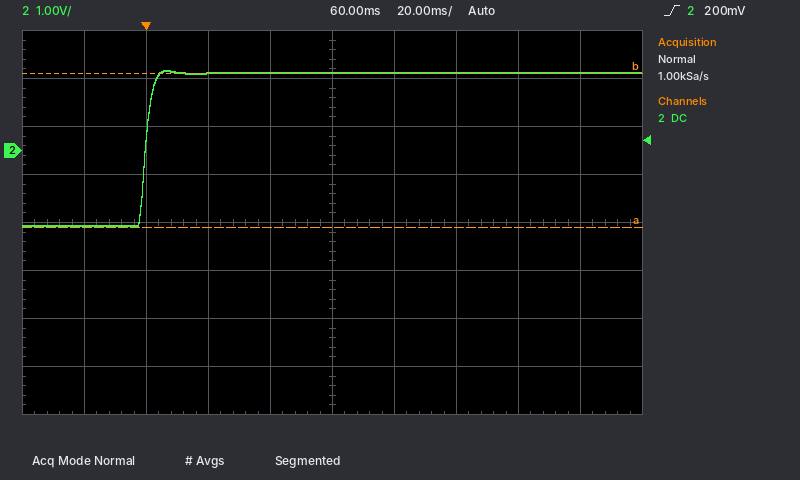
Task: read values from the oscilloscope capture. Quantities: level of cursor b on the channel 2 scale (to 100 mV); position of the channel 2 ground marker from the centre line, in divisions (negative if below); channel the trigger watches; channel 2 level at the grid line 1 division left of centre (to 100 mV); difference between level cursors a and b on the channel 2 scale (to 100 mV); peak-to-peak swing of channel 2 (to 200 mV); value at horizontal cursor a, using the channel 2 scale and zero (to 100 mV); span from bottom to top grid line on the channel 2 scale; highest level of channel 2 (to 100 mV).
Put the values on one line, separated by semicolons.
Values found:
1.6 V; +1.5 div; channel 2; 1.6 V; 3.2 V; 3.2 V; -1.6 V; 8 V; 1.7 V
